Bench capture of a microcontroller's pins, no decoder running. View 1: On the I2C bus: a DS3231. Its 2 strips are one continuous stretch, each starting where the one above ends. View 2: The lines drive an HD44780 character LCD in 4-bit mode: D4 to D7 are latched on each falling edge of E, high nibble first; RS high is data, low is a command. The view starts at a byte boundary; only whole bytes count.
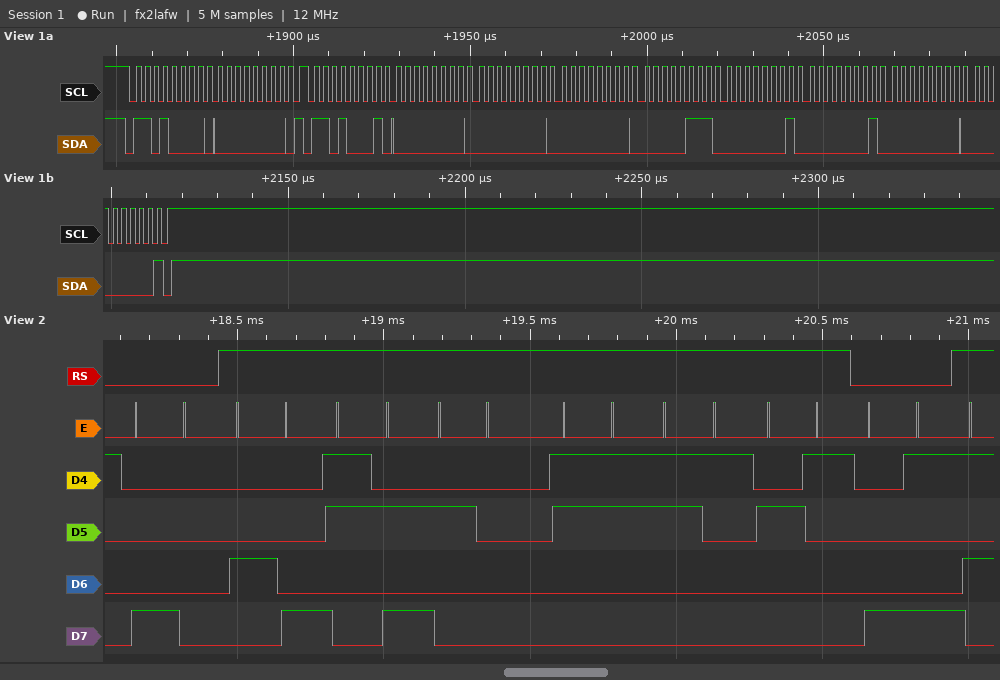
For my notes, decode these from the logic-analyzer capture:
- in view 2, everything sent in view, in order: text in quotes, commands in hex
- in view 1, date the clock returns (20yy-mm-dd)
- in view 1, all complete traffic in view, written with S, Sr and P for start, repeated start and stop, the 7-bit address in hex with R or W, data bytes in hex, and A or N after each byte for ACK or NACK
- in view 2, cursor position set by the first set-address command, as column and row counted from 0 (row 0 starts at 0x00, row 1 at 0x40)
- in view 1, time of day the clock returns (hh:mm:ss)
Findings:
0x80 "H: 31!" 0x89
2000-01-01
S 68W A 00 A Sr 68R A 00 A 00 A 00 A 07 A 01 A 01 A 00 A 00 N P
column 0, row 0
00:00:00
